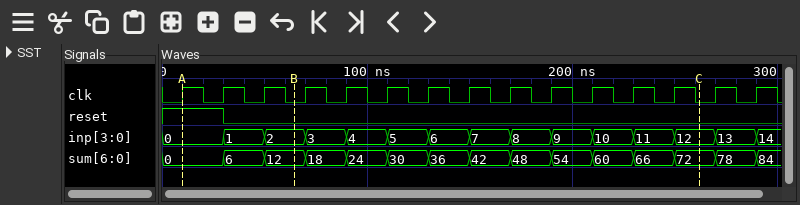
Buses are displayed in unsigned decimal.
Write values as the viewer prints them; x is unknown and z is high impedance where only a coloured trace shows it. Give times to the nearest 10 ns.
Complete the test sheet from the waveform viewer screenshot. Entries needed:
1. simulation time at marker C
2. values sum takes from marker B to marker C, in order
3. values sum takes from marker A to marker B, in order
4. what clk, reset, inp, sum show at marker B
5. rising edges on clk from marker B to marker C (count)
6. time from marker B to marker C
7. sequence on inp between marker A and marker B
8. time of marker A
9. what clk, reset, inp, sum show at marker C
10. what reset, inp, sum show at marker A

260 ns
12, 18, 24, 30, 36, 42, 48, 54, 60, 66, 72
0, 6, 12
clk=0, reset=0, inp=2, sum=12
10
200 ns
0, 1, 2
10 ns
clk=0, reset=0, inp=12, sum=72
reset=1, inp=0, sum=0
